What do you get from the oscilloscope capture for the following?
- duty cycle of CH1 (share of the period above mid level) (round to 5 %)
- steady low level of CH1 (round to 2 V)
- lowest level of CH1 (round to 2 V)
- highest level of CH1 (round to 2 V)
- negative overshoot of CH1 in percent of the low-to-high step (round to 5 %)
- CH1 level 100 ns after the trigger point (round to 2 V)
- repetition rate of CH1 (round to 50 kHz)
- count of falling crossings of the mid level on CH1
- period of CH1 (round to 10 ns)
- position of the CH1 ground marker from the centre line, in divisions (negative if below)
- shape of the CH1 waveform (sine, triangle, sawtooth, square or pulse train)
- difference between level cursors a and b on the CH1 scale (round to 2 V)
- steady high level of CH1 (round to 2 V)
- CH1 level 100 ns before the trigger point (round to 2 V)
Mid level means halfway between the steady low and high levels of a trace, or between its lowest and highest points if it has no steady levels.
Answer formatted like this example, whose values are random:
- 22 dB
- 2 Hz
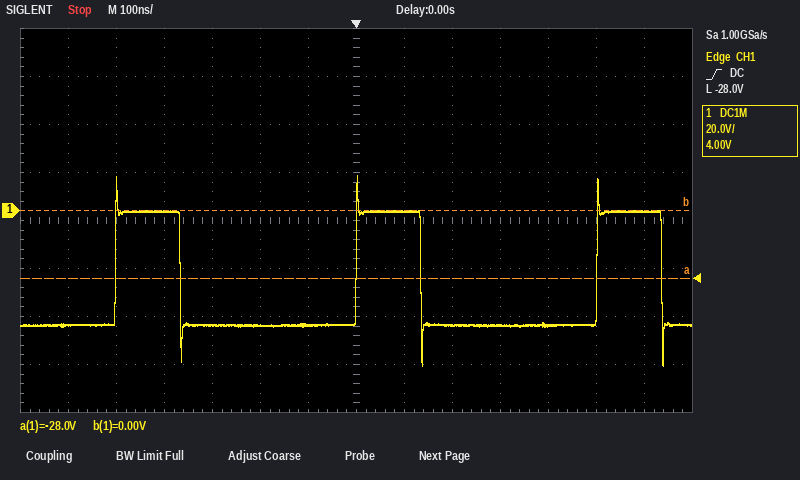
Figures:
- 25 %
- -48 V
- -64 V
- 14 V
- 35 %
- 0 V
- 2.00 MHz
- 3
- 500 ns
- +0.2 div
- pulse train
- 28 V
- 0 V
- -48 V
